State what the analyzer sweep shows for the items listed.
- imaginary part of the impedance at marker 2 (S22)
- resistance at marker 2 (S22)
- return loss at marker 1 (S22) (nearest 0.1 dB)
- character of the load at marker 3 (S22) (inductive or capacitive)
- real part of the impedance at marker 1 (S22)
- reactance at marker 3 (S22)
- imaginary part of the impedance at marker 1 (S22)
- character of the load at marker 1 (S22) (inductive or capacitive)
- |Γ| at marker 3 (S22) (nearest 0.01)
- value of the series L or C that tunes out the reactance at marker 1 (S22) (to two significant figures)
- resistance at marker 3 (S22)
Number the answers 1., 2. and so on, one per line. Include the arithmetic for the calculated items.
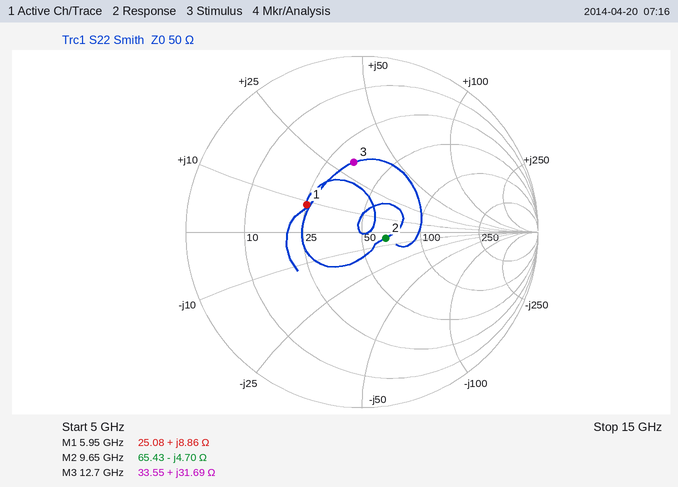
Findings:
1. -4.70 Ω
2. 65.43 Ω
3. 9.1 dB
4. inductive
5. 25.08 Ω
6. +31.69 Ω
7. +8.86 Ω
8. inductive
9. 0.40
10. C = 1/(2π × 5.95 GHz × 8.86 Ω) ≈ 3.0 pF
11. 33.55 Ω
